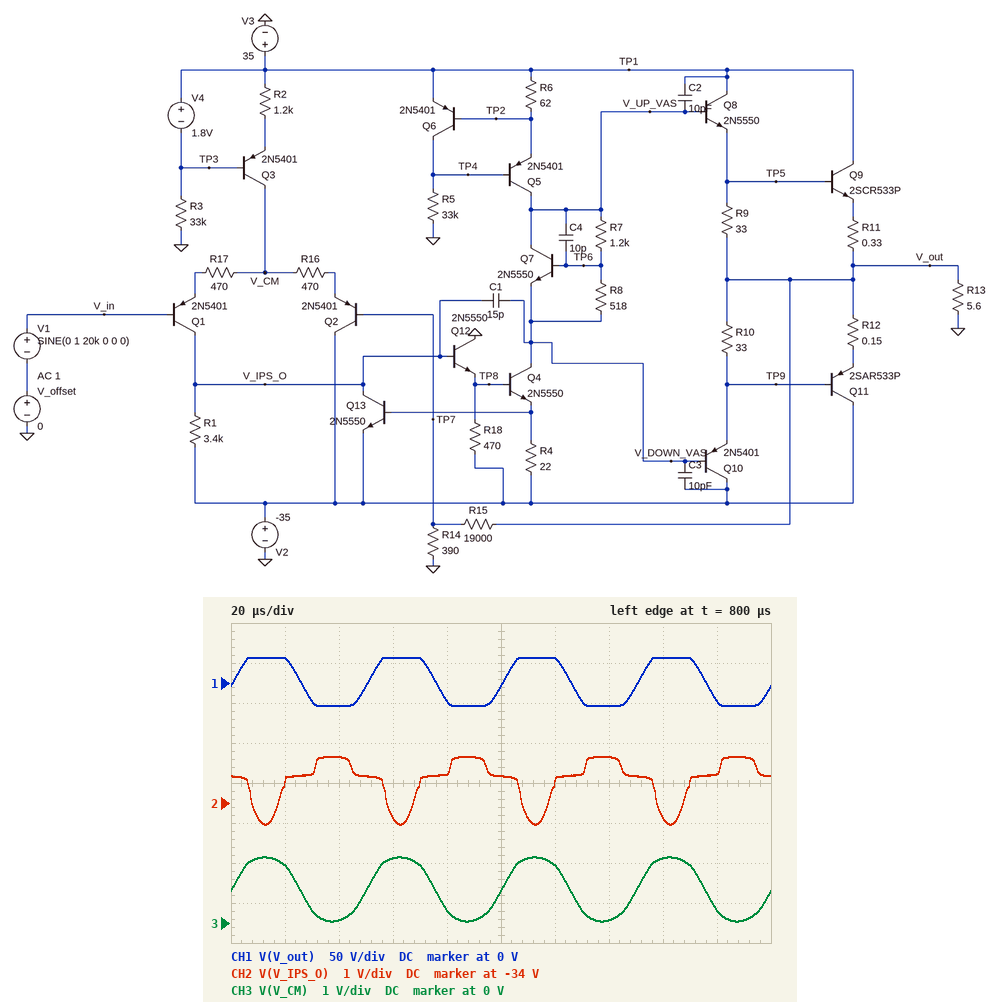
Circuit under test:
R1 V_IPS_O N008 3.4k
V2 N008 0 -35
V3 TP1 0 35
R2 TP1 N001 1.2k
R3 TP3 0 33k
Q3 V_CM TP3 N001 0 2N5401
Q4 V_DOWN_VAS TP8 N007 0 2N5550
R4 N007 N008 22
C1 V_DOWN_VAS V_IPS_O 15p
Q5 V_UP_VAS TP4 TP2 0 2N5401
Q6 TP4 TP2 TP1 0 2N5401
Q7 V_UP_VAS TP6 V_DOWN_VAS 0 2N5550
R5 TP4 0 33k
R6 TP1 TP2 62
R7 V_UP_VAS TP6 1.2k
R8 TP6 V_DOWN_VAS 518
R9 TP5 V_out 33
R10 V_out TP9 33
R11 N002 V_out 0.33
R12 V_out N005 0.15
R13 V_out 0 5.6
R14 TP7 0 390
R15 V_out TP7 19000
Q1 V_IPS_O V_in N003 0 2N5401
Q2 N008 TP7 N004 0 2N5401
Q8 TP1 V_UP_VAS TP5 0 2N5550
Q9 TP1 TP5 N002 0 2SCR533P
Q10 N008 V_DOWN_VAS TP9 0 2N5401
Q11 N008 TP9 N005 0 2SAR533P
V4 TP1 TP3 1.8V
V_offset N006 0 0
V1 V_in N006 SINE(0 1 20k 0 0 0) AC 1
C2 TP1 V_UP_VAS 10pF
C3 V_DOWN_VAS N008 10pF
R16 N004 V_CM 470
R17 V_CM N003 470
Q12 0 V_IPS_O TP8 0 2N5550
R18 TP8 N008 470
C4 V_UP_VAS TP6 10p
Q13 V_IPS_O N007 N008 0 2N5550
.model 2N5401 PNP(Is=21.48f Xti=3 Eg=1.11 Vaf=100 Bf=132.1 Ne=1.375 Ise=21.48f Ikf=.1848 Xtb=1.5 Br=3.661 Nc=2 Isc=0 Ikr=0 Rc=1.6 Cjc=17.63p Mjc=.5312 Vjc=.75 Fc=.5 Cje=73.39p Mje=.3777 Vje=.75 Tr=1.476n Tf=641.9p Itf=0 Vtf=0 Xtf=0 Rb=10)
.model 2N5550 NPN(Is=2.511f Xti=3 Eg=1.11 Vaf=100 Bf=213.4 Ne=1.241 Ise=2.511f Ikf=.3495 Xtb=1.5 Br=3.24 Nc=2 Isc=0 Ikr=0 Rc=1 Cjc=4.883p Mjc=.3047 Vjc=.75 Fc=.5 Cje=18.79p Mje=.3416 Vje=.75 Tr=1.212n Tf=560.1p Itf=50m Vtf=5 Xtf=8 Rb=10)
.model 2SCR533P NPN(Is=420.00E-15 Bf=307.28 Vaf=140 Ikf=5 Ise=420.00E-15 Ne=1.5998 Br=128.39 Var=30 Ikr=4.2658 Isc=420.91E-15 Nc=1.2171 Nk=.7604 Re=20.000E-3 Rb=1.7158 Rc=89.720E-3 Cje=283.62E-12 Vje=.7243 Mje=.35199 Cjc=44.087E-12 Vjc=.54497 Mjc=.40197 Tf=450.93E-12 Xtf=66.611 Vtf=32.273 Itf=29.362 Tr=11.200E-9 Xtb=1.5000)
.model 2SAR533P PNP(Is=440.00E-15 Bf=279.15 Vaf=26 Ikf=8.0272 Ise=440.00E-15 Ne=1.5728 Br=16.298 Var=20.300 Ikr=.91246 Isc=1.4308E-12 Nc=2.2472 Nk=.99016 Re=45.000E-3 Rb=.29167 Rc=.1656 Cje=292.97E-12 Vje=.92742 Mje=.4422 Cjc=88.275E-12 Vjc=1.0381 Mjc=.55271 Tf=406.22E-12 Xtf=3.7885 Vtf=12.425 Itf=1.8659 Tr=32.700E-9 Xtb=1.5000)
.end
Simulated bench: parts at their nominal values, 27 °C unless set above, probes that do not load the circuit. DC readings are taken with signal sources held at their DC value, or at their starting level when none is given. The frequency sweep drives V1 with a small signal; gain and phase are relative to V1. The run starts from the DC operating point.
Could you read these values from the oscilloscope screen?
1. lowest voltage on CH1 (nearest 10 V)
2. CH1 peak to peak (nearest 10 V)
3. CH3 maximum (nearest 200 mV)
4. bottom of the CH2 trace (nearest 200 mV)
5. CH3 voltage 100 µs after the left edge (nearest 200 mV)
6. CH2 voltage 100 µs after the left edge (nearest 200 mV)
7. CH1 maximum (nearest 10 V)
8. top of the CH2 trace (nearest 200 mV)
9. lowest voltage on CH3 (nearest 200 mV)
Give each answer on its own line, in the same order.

-30 V
60 V
1.6 V
-34.6 V
800 mV
-33.4 V
30 V
-32.8 V
0 V
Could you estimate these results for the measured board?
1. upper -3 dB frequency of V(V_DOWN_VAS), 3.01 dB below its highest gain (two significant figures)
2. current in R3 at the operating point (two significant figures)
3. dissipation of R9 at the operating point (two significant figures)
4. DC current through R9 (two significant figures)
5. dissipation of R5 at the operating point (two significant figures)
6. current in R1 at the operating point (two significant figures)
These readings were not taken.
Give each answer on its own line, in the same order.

190 kHz
1.0 mA
18 mW
23 mA
34 mW
490 µA
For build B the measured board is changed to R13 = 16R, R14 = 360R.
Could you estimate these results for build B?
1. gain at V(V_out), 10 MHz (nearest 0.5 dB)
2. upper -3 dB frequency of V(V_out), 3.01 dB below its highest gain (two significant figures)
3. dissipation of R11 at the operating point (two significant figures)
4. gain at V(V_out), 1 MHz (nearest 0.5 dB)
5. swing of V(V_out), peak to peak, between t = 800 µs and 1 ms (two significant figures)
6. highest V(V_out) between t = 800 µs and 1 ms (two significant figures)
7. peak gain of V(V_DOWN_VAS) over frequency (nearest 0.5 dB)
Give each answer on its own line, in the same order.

-0.5 dB
180 kHz
2.0 mW
19.5 dB
65 V
33 V
35.0 dB
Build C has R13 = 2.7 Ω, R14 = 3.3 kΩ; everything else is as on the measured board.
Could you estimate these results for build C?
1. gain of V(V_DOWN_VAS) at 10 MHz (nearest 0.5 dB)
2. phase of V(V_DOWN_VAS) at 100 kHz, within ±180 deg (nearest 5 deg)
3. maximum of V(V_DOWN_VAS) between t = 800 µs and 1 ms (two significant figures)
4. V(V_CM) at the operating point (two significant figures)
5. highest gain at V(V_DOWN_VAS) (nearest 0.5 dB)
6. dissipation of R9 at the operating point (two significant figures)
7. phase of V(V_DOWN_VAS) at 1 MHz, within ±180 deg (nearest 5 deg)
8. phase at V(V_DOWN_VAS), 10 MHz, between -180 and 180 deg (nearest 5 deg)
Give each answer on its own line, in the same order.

-4.5 dB
-5 deg
6.8 V
850 mV
19.5 dB
13 mW
-50 deg
-145 deg
